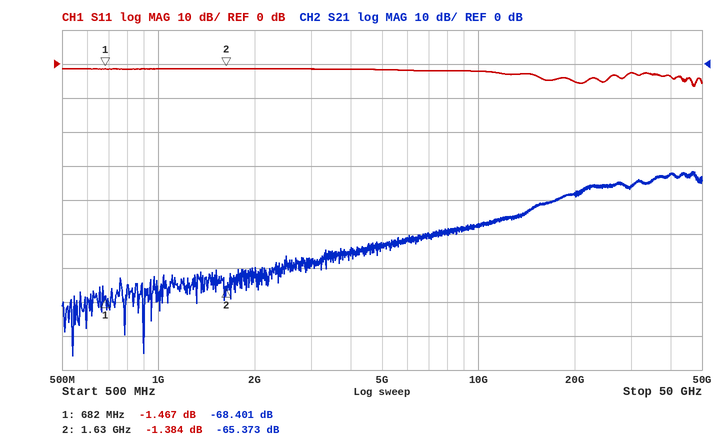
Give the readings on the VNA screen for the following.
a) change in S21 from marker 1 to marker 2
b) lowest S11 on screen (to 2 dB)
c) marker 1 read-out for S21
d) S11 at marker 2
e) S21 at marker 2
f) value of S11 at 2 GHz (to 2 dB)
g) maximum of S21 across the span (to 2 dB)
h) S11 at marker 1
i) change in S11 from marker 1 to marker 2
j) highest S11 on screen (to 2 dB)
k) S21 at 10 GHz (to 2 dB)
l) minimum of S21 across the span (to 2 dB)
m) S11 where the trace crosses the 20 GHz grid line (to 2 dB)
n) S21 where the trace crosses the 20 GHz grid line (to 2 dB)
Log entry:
3.028 dB
-6 dB
-68.401 dB
-1.384 dB
-65.373 dB
-2 dB
-32 dB
-1.467 dB
0.083 dB
-2 dB
-48 dB
-86 dB
-6 dB
-38 dB
